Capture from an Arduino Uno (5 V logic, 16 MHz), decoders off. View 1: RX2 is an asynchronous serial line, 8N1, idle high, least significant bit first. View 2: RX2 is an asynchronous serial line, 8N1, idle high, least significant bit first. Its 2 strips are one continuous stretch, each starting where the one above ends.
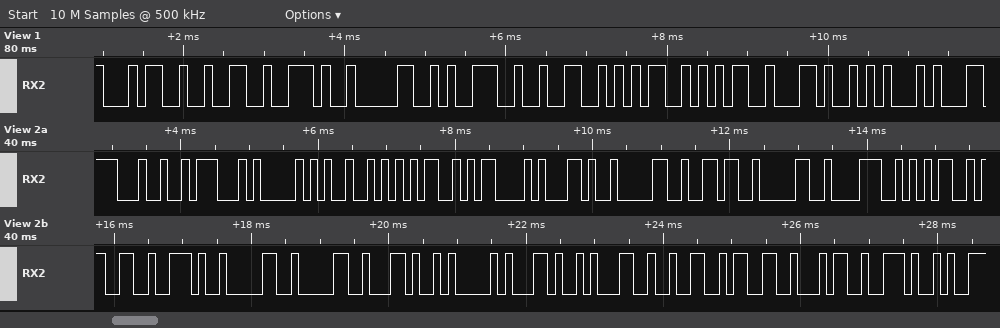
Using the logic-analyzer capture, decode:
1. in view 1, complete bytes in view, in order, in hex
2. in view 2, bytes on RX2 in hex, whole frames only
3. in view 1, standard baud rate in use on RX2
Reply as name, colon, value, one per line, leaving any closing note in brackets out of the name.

in view 1, complete bytes in view, in order, in hex: 34 32 2E 30 39 32 35 35 2C 45
in view 2, bytes on RX2 in hex, whole frames only: 24 47 50 52 4D 43 2C 30 36 30 38 35 33 2E 30 30 2C 41 2C 31 32 33 34 2E
in view 1, standard baud rate in use on RX2: 9600 baud
